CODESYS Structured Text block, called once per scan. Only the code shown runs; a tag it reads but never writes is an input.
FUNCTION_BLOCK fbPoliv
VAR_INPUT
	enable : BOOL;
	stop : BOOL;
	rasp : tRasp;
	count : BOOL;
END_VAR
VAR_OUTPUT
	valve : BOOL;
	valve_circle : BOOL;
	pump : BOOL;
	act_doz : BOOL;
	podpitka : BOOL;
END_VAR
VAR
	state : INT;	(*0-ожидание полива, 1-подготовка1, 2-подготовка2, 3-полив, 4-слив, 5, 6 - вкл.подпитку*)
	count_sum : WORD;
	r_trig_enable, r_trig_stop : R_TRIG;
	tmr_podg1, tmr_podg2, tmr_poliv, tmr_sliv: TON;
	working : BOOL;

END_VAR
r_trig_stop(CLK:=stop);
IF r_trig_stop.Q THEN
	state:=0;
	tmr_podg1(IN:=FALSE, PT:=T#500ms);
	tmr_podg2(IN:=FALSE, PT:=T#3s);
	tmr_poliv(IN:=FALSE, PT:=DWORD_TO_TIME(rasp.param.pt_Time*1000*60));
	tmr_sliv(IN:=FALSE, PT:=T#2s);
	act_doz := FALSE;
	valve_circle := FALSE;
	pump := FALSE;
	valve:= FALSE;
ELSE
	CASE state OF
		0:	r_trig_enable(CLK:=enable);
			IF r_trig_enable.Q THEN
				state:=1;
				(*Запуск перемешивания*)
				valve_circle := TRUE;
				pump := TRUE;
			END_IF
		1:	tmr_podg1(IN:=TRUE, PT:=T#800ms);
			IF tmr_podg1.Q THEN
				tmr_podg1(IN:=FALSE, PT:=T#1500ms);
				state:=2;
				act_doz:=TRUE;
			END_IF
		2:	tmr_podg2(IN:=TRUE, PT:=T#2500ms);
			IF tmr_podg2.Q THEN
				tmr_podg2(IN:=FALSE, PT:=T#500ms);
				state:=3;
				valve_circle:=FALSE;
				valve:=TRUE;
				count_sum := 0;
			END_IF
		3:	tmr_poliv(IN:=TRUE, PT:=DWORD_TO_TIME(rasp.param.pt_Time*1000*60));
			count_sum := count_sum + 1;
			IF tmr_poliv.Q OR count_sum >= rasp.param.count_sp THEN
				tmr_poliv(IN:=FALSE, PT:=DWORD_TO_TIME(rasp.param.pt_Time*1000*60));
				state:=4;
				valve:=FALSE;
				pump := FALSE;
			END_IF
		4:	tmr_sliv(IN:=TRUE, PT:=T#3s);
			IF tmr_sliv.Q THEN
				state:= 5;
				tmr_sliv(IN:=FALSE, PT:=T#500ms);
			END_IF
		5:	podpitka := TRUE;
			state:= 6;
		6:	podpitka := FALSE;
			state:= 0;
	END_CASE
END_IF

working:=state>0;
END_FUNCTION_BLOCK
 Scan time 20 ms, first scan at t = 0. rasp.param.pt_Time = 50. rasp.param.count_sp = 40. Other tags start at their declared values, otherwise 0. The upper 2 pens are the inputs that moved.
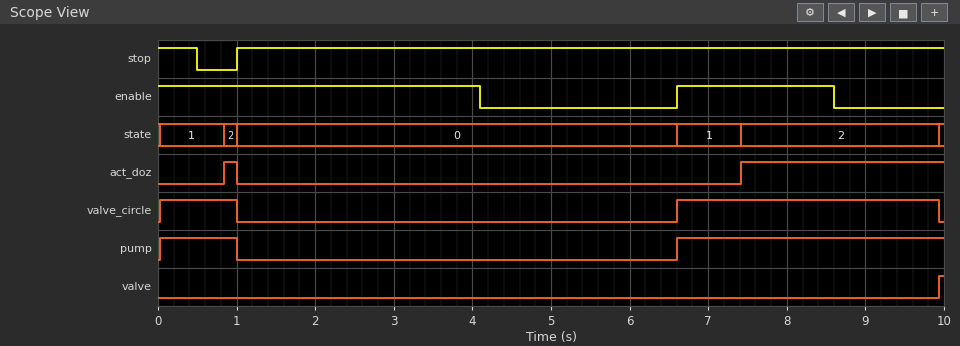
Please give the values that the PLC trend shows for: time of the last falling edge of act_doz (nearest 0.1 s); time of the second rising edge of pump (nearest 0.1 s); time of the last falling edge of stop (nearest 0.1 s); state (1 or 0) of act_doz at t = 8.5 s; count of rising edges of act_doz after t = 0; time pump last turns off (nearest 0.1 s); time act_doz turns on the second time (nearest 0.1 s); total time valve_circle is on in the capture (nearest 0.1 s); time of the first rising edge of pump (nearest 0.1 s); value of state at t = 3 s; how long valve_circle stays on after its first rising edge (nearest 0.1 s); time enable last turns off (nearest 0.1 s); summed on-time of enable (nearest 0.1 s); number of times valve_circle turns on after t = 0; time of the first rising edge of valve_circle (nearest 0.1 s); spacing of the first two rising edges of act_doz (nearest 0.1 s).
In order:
1.0 s
6.6 s
0.5 s
1
2
1.0 s
7.4 s
4.3 s
0.0 s
0
1.0 s
8.6 s
6.1 s
2
0.0 s
6.6 s
